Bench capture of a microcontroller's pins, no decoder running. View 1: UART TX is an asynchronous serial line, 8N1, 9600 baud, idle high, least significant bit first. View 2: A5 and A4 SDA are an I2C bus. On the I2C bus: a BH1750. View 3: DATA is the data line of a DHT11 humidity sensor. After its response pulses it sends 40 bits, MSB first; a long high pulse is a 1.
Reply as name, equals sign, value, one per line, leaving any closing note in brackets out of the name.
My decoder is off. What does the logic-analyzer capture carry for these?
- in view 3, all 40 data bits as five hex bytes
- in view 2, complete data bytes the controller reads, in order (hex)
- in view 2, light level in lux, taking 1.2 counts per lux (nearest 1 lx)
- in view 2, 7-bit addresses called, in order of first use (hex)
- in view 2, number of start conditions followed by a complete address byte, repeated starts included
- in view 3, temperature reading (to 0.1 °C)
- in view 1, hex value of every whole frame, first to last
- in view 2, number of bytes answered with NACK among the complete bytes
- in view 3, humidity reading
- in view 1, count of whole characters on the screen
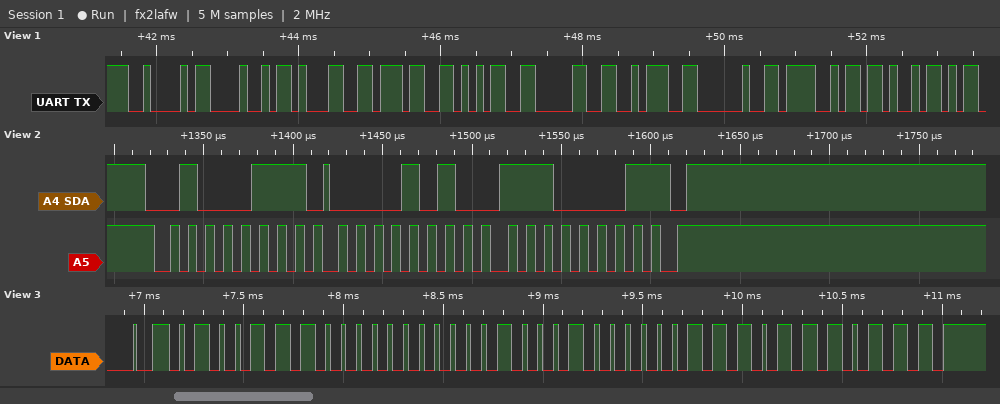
in view 3, all 40 data bits as five hex bytes = 4E 00 22 07 77
in view 2, complete data bytes the controller reads, in order = 0A E1
in view 2, light level in lux, taking 1.2 counts per lux = 2321 lx
in view 2, 7-bit addresses called, in order of first use = 0x23
in view 2, number of start conditions followed by a complete address byte, repeated starts included = 1
in view 3, temperature reading = 34.7 °C
in view 1, hex value of every whole frame, first to last = 0x42 0x48 0x31 0x37 0x35 0x30 0x3A 0x20 0x4F 0x4B
in view 2, number of bytes answered with NACK among the complete bytes = 1
in view 3, humidity reading = 78 %
in view 1, count of whole characters on the screen = 10
